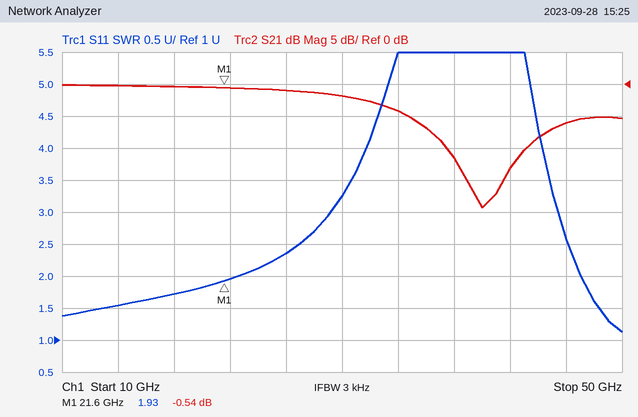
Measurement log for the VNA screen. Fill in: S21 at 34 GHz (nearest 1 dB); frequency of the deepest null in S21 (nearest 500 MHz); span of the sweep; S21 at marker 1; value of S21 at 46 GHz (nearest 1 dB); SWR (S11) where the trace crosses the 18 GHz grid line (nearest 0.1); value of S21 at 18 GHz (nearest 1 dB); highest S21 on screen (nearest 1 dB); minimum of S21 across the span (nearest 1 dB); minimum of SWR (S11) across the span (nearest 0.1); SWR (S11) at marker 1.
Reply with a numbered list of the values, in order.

1. -4 dB
2. 40.0 GHz
3. 40 GHz
4. -0.54 dB
5. -6 dB
6. 1.7
7. 0 dB
8. 0 dB
9. -19 dB
10. 1.1
11. 1.93
